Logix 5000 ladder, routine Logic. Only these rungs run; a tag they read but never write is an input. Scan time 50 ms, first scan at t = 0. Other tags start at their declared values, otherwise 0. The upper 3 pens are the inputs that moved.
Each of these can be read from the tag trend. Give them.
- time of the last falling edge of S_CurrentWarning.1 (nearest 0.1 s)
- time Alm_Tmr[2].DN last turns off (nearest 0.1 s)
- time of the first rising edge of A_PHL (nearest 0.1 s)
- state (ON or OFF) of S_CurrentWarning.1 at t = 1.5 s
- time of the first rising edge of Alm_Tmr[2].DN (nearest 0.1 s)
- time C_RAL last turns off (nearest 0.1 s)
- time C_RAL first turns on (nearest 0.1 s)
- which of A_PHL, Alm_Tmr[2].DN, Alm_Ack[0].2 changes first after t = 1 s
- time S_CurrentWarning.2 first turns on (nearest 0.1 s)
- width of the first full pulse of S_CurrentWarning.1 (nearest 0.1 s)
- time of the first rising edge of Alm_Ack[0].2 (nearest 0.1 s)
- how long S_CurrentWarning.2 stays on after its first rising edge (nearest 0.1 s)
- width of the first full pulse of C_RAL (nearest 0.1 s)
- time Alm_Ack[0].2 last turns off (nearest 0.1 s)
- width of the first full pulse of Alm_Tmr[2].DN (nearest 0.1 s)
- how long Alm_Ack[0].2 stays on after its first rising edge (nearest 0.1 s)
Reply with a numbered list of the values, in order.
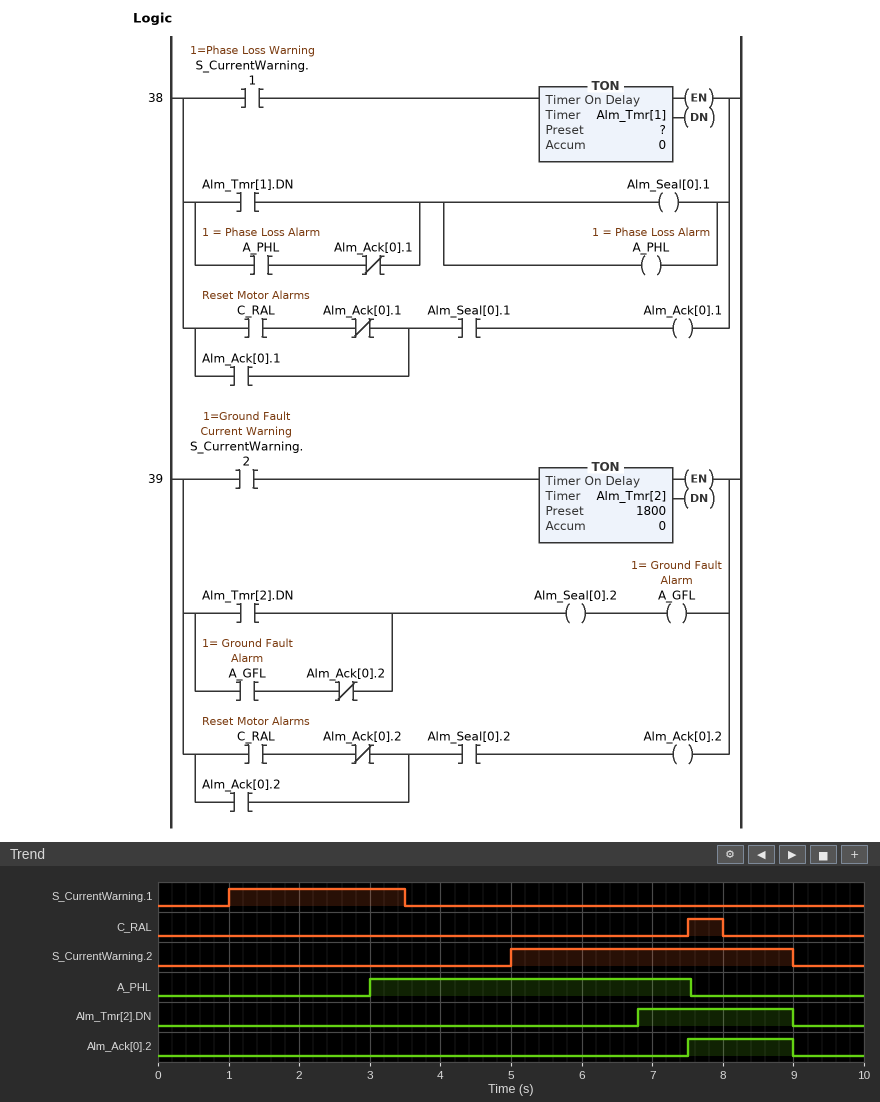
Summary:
1. 3.5 s
2. 9.0 s
3. 3.0 s
4. ON
5. 6.8 s
6. 8.0 s
7. 7.5 s
8. A_PHL
9. 5.0 s
10. 2.5 s
11. 7.5 s
12. 4.0 s
13. 0.5 s
14. 9.0 s
15. 2.2 s
16. 1.5 s
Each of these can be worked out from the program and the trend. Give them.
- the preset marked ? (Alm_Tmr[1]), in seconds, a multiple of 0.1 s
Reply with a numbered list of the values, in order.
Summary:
1. 2.0 s
